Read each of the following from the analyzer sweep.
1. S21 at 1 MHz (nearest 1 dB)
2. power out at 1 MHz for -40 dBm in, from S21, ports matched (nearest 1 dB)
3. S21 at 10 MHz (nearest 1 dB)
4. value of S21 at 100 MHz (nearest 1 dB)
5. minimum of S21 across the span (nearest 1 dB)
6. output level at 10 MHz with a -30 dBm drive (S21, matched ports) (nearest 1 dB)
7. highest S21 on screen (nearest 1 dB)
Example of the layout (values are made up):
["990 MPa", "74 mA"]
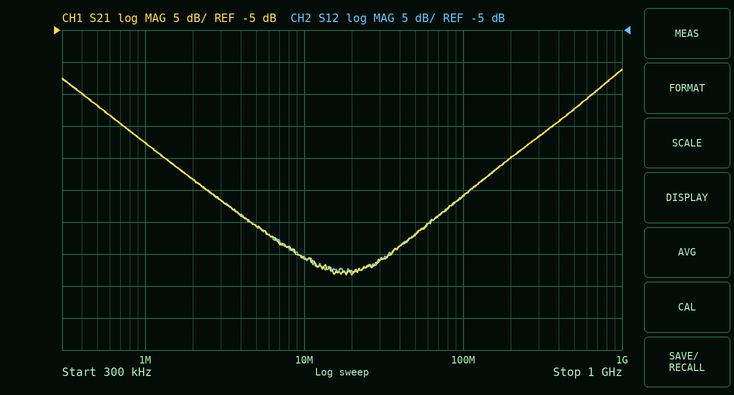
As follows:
["-23 dB", "-63 dBm", "-41 dB", "-31 dB", "-43 dB", "-71 dBm", "-11 dB"]
